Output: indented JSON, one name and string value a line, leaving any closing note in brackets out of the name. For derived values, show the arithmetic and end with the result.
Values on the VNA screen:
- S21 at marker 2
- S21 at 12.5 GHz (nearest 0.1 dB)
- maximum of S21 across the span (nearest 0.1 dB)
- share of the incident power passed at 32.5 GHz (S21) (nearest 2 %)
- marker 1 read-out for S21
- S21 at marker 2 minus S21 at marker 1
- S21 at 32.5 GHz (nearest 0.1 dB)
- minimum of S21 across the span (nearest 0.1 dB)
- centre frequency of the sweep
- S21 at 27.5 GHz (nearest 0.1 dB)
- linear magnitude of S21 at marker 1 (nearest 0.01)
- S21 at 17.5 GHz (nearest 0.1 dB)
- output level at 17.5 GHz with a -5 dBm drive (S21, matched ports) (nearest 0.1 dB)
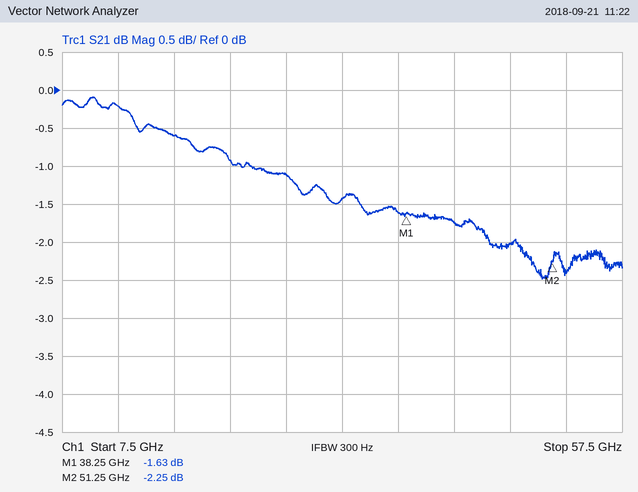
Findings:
{
  "S21 at marker 2": "-2.25 dB",
  "S21 at 12.5 GHz": "-0.2 dB",
  "maximum of S21 across the span": "-0.1 dB",
  "share of the incident power passed at 32.5 GHz (S21)": "10^(-1.4/10) ≈ 72 %",
  "marker 1 read-out for S21": "-1.63 dB",
  "S21 at marker 2 minus S21 at marker 1": "-2.25 − (-1.63) = -0.62 dB",
  "S21 at 32.5 GHz": "-1.4 dB",
  "minimum of S21 across the span": "-2.5 dB",
  "centre frequency of the sweep": "32.5 GHz",
  "S21 at 27.5 GHz": "-1.1 dB",
  "linear magnitude of S21 at marker 1": "10^(-1.63/20) ≈ 0.83",
  "S21 at 17.5 GHz": "-0.6 dB",
  "output level at 17.5 GHz with a -5 dBm drive (S21, matched ports)": "-5 dBm + (-0.6 dB) = -5.6 dBm"
}
